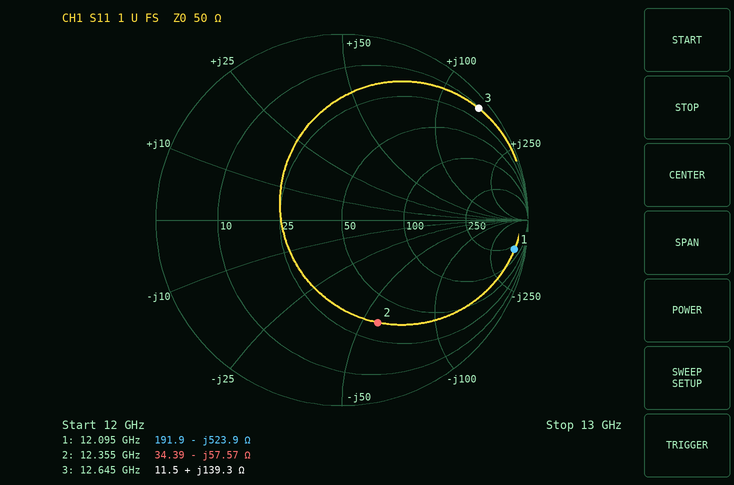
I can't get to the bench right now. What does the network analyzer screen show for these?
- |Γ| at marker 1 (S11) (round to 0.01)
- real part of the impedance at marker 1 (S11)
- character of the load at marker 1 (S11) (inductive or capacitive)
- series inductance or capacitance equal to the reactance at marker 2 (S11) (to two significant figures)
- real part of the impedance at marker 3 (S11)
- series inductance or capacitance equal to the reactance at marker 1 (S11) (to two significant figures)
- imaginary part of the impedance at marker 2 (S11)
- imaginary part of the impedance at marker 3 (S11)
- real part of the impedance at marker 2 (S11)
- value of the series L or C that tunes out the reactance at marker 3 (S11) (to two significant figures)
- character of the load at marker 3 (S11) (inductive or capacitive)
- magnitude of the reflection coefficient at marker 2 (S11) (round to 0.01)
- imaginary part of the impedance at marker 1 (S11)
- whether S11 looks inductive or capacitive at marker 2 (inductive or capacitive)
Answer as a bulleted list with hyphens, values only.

- 0.94
- 191.9 Ω
- capacitive
- 220 fF
- 11.5 Ω
- 25 fF
- -57.57 Ω
- +139.3 Ω
- 34.39 Ω
- 90 fF
- inductive
- 0.58
- -523.9 Ω
- capacitive
